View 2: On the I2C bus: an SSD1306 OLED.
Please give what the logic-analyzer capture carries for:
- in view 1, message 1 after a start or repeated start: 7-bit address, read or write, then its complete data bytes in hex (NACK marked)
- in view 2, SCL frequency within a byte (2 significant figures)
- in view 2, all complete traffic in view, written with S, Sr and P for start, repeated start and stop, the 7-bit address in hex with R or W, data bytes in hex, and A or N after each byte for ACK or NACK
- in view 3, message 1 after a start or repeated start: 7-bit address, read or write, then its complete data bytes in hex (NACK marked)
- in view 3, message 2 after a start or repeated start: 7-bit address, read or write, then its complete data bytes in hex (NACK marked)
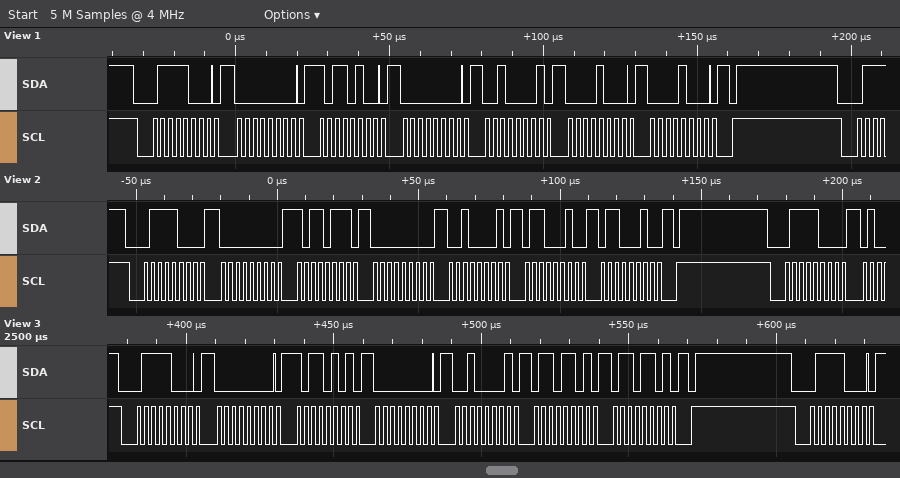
0x3C write: 00 B4 00 21 08 08
400 kHz
S 3CW A 00 A B7 A 00 A 21 A 62 A 62 A P S 3CW A
0x3C write: 00 B5 00 21 6D 6D
0x3C write
